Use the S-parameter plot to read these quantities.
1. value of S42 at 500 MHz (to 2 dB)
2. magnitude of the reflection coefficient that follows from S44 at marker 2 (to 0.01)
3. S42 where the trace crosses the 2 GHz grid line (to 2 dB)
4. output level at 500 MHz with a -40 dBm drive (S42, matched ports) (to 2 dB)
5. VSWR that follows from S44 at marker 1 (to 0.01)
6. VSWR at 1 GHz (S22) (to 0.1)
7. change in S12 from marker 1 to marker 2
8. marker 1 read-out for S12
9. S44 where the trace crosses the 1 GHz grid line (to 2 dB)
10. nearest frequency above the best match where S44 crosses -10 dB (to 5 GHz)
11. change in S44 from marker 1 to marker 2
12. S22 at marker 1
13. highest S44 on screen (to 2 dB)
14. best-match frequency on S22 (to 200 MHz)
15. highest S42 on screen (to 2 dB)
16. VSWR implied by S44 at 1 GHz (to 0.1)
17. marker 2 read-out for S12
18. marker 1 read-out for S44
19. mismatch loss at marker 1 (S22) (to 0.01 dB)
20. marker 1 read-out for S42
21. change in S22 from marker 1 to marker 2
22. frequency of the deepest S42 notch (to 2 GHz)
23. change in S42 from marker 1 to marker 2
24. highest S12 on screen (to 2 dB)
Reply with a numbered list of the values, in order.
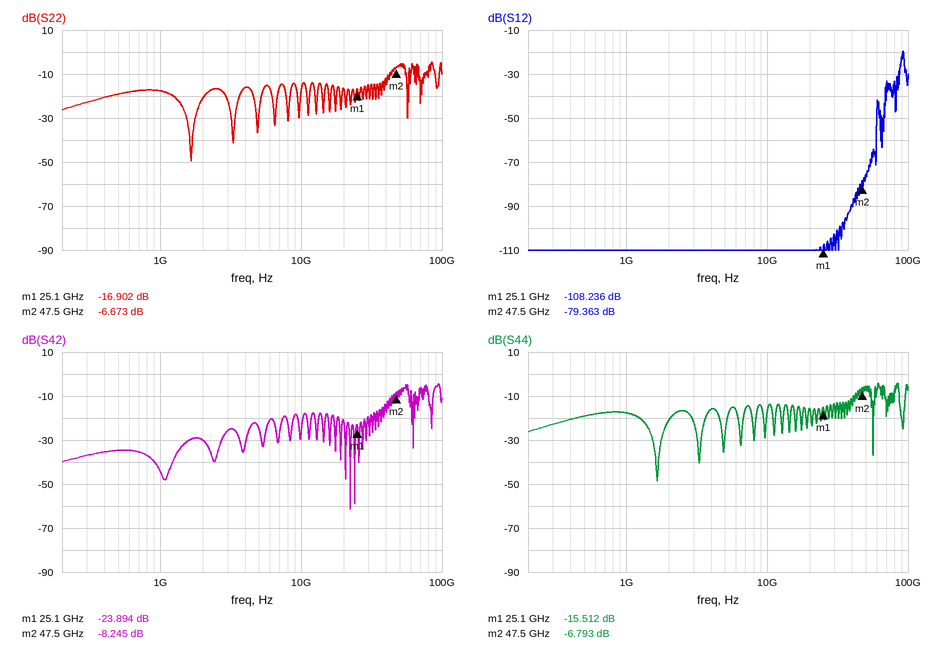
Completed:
1. -34 dB
2. 0.46
3. -30 dB
4. -74 dBm
5. 1.40
6. 1.3
7. 28.873 dB
8. -108.236 dB
9. -18 dB
10. 40 GHz
11. 8.719 dB
12. -16.902 dB
13. -4 dB
14. 1.6 GHz
15. -4 dB
16. 1.3
17. -79.363 dB
18. -15.512 dB
19. 0.09 dB
20. -23.894 dB
21. 10.229 dB
22. 22 GHz
23. 15.649 dB
24. -20 dB
